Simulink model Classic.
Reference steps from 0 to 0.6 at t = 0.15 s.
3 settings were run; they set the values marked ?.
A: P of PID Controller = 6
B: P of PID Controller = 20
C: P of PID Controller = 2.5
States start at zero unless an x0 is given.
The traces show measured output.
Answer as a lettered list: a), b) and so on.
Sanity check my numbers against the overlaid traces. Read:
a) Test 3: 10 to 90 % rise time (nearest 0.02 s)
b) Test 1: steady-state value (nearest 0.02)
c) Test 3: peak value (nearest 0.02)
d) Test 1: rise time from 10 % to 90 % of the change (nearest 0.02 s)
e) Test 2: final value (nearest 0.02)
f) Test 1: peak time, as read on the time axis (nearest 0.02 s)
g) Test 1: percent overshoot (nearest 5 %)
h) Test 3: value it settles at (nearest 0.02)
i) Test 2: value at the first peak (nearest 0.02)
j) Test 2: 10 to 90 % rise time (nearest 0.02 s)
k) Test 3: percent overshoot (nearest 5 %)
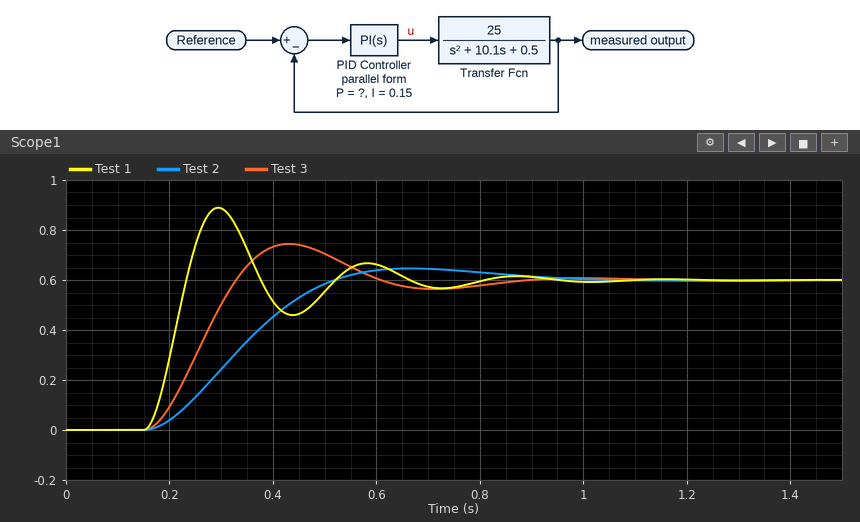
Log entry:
a) 0.12 s
b) 0.60
c) 0.74
d) 0.06 s
e) 0.60
f) 0.30 s
g) 50 %
h) 0.60
i) 0.64
j) 0.24 s
k) 25 %
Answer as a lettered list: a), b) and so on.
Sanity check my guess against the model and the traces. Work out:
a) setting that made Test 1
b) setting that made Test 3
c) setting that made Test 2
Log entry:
a) B
b) A
c) C
